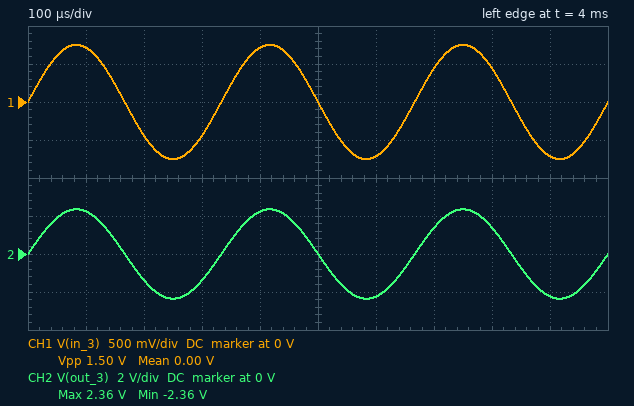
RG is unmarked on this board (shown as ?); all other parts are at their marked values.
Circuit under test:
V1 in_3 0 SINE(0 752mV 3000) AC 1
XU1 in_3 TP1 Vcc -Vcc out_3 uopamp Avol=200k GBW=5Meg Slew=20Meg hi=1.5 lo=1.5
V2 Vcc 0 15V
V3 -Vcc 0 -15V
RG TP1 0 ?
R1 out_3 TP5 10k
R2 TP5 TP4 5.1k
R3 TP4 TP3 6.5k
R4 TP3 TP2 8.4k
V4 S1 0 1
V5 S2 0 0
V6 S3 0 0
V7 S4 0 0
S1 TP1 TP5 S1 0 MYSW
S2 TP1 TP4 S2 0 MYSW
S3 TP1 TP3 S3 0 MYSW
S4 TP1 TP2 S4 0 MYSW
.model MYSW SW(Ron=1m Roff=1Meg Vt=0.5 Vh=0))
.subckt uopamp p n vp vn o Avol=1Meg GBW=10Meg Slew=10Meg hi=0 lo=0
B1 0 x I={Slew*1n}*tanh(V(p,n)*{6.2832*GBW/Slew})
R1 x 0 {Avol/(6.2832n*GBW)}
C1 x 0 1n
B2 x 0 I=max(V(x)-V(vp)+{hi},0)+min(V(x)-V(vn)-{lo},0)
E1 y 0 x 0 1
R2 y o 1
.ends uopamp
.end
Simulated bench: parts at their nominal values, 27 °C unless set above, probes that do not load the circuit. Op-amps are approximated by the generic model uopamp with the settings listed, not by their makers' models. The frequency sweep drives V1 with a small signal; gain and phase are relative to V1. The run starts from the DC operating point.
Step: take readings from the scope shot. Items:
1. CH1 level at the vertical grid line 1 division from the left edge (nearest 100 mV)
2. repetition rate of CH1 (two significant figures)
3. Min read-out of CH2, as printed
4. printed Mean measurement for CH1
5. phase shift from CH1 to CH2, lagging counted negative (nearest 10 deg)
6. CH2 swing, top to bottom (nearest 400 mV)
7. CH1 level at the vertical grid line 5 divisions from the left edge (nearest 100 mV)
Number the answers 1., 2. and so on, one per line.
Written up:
1. 700 mV
2. 3.0 kHz
3. -2.36 V
4. 0.00 V
5. 0 deg
6. 4.8 V
7. 0 V
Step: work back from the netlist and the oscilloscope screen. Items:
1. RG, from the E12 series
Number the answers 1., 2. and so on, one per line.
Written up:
1. 4.7 kΩ
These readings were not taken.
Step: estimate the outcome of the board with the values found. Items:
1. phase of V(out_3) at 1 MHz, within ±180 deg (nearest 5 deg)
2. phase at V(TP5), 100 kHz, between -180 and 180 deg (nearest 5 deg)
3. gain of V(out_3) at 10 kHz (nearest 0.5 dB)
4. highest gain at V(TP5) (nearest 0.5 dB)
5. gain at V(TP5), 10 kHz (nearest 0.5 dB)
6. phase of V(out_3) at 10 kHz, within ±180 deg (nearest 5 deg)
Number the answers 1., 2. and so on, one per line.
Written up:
1. -85 deg
2. -50 deg
3. 35.0 dB
4. 35.0 dB
5. 35.0 dB
6. -5 deg
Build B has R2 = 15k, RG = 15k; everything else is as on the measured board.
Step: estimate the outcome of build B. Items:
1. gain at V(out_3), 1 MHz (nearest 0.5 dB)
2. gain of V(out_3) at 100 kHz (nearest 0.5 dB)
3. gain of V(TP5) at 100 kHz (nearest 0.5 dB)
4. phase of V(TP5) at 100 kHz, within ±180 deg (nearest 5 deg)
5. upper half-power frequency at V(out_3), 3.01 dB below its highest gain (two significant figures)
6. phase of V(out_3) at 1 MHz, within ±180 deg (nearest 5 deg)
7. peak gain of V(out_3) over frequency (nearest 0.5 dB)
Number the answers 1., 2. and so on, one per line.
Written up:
1. 13.5 dB
2. 25.0 dB
3. 24.5 dB
4. -20 deg
5. 260 kHz
6. -75 deg
7. 25.5 dB
